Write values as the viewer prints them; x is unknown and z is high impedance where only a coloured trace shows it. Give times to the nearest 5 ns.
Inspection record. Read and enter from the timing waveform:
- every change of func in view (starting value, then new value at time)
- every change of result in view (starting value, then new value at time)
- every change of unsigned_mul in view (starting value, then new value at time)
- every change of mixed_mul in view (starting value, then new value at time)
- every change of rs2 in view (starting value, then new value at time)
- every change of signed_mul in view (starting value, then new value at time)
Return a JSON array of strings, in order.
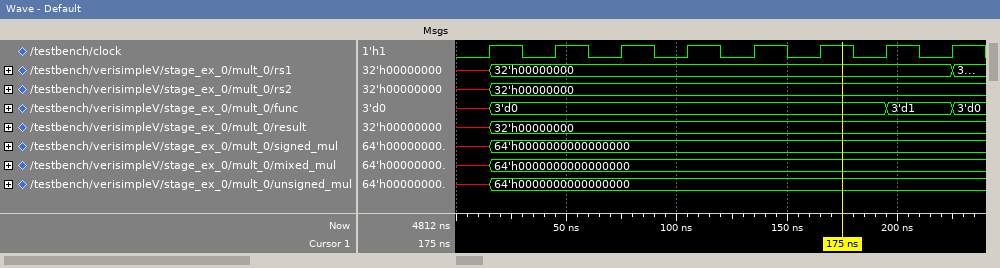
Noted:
["x, 3'd0 at 15 ns, 3'd1 at 195 ns, 3'd0 at 225 ns", "x, 32'h00000000 at 15 ns", "x, 64'h0000000000000000 at 15 ns", "x, 64'h0000000000000000 at 15 ns", "x, 32'h00000000 at 15 ns", "x, 64'h0000000000000000 at 15 ns"]
